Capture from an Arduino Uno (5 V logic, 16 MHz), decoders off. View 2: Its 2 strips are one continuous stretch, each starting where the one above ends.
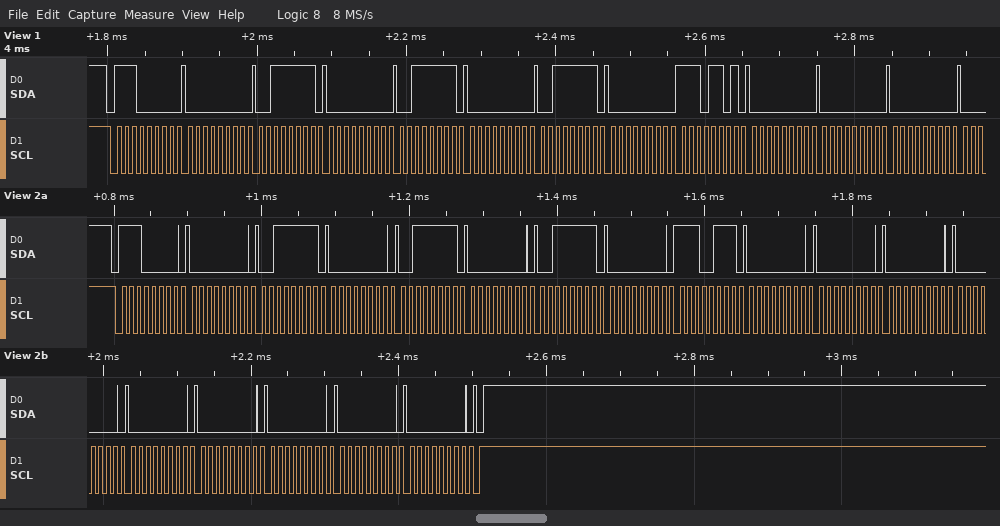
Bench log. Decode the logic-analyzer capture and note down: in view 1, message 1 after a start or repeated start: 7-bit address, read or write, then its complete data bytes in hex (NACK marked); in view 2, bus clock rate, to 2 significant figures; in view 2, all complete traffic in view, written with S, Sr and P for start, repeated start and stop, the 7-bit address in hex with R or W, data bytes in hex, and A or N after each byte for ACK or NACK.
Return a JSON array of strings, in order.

["0x70 write: 00 3F 00 3F 00 3F 00 ED 00 00 00", "100 kHz", "S 70W A 00 A 3F A 00 A 3F A 00 A 3F A 00 A E7 A 00 A 00 A 00 A 00 A 00 A 00 A 00 A 00 A 00 A P"]
